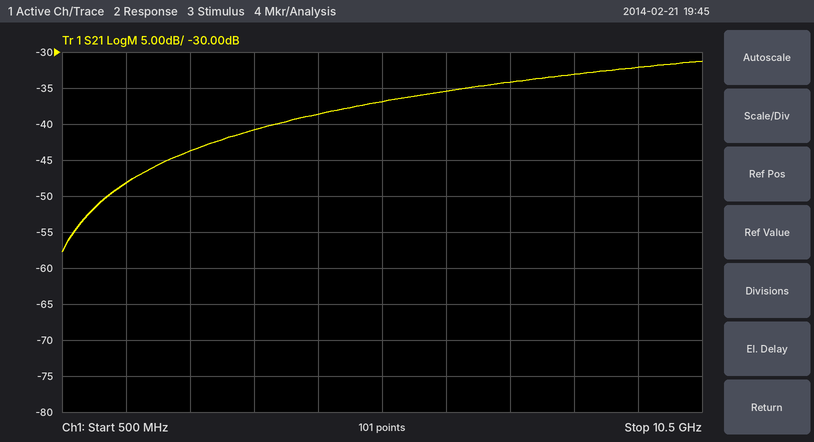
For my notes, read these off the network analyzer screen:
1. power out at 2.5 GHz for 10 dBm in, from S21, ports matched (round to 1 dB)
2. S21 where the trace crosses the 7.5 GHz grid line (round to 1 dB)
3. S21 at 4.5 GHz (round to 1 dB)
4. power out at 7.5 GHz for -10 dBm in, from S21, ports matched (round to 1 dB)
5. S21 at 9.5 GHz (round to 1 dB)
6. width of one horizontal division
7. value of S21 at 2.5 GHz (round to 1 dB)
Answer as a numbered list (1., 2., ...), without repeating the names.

1. -34 dBm
2. -34 dB
3. -39 dB
4. -44 dBm
5. -32 dB
6. 1 GHz
7. -44 dB
